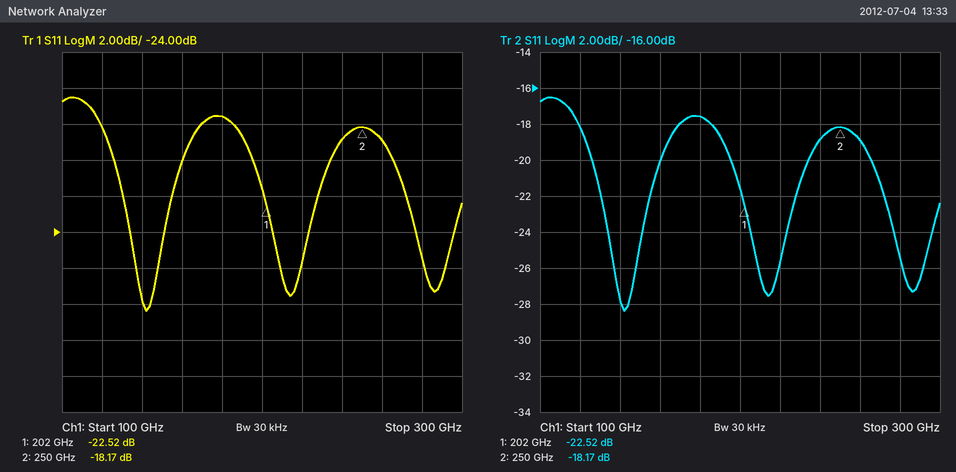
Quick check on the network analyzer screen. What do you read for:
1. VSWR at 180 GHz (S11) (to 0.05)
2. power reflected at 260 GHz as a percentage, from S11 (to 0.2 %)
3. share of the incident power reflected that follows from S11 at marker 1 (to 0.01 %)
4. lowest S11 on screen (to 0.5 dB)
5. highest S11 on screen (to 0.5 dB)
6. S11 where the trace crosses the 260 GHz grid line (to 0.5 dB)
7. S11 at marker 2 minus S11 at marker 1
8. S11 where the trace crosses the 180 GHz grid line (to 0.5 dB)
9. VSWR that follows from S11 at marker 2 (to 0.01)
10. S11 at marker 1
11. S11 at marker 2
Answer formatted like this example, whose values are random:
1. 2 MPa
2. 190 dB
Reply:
1. 1.30
2. 1.2 %
3. 0.56 %
4. -28.5 dB
5. -16.5 dB
6. -19.0 dB
7. 4.35 dB
8. -17.5 dB
9. 1.28
10. -22.52 dB
11. -18.17 dB
